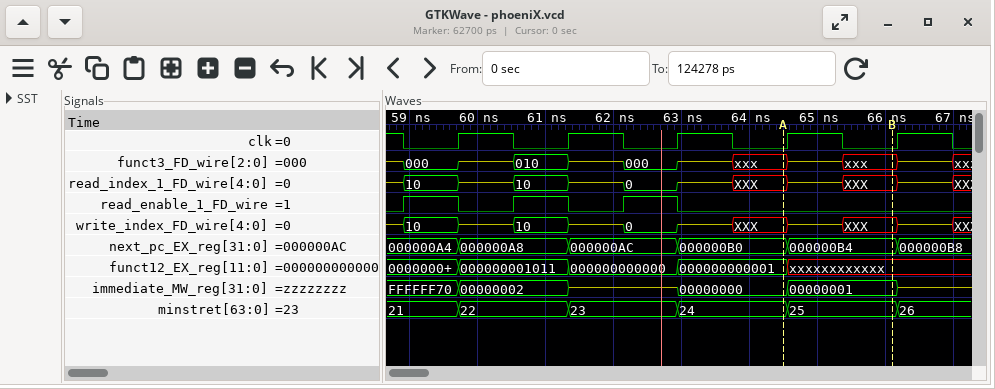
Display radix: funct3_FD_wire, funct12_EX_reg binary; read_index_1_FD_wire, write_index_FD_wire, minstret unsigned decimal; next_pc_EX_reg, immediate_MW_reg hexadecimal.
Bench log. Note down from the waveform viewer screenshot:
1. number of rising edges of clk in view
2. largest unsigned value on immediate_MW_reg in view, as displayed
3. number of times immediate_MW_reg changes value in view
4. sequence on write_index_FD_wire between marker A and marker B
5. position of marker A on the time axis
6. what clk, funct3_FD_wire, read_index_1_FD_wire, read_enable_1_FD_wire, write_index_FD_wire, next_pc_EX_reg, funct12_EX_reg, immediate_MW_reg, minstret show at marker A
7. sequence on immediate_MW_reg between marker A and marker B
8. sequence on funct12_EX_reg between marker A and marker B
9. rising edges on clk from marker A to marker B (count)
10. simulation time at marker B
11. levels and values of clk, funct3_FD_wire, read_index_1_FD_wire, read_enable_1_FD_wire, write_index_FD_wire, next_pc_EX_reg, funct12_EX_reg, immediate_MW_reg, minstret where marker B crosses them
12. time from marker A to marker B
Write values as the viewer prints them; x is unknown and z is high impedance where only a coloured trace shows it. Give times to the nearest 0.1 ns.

5
FFFFFF70
5
XXX, z, XXX
64.5 ns
clk=0, funct3_FD_wire=xxx, read_index_1_FD_wire=XXX, read_enable_1_FD_wire=0, write_index_FD_wire=XXX, next_pc_EX_reg=000000B0, funct12_EX_reg=000000000001, immediate_MW_reg=00000000, minstret=24
00000000, 00000001
000000000001, xxxxxxxxxxxx
1
66.1 ns
clk=0, funct3_FD_wire=xxx, read_index_1_FD_wire=XXX, read_enable_1_FD_wire=0, write_index_FD_wire=XXX, next_pc_EX_reg=000000B4, funct12_EX_reg=xxxxxxxxxxxx, immediate_MW_reg=00000001, minstret=25
1.6 ns
